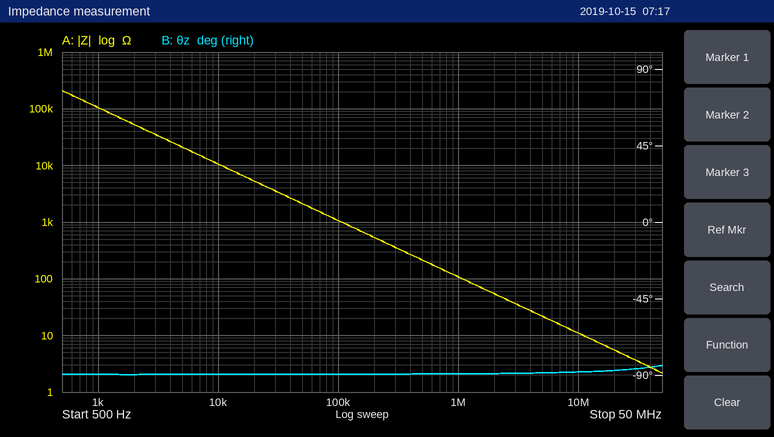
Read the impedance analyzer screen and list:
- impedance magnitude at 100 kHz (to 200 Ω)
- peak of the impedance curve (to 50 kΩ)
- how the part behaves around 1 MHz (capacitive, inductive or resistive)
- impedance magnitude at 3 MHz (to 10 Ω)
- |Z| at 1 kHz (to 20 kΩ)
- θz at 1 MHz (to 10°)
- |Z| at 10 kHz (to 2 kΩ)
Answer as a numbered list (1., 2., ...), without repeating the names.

1. 1.0 kΩ
2. 200 kΩ
3. capacitive
4. 40 Ω
5. 100 kΩ
6. -90°
7. 10 kΩ
